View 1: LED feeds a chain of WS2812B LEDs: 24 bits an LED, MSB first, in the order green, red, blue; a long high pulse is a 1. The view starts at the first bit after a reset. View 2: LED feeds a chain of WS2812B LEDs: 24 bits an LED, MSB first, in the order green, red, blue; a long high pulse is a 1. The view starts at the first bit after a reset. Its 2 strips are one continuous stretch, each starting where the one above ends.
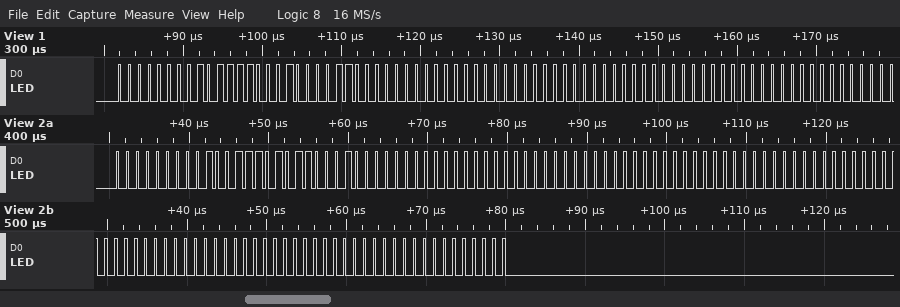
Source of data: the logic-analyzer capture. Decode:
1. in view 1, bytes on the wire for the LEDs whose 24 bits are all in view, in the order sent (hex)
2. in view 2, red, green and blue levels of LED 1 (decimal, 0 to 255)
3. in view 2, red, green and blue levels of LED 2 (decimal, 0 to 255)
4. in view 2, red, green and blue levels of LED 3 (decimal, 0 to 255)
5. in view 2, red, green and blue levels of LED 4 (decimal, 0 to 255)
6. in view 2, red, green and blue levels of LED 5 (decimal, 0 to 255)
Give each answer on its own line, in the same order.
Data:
00 BC 43 00 00 00 00 00 00
78, 0, 177
0, 0, 0
0, 0, 0
0, 0, 0
0, 0, 0
